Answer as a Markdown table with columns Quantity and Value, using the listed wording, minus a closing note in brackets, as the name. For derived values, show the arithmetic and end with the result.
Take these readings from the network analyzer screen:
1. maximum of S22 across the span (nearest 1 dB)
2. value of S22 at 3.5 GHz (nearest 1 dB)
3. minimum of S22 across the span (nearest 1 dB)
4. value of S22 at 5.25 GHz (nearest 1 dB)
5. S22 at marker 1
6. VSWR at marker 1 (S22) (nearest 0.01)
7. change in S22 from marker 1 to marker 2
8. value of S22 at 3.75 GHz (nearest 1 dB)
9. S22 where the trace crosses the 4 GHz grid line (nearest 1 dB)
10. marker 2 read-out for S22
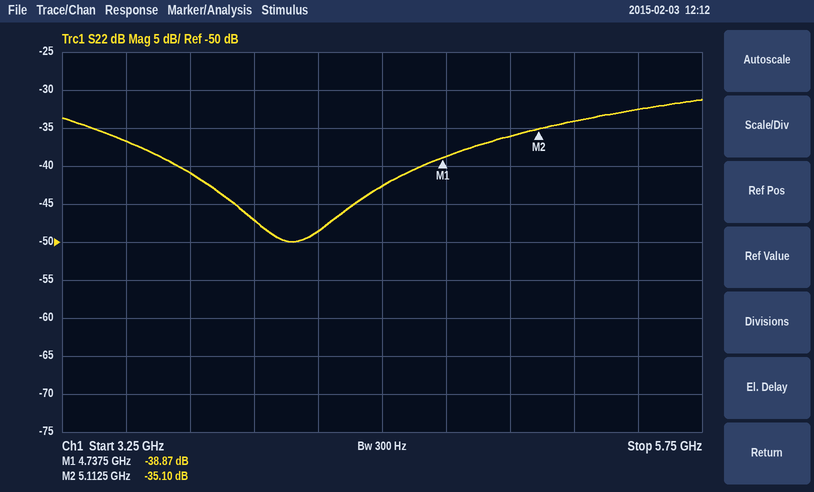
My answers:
| Quantity | Value |
|---|---|
| maximum of S22 across the span | -31 dB |
| value of S22 at 3.5 GHz | -37 dB |
| minimum of S22 across the span | -50 dB |
| value of S22 at 5.25 GHz | -34 dB |
| S22 at marker 1 | -38.87 dB |
| VSWR at marker 1 (S22) | (1 + 0.0114)/(1 − 0.0114) ≈ 1.02 |
| change in S22 from marker 1 to marker 2 | -35.1 − (-38.87) = 3.77 dB |
| value of S22 at 3.75 GHz | -41 dB |
| S22 where the trace crosses the 4 GHz grid line | -47 dB |
| marker 2 read-out for S22 | -35.10 dB |
